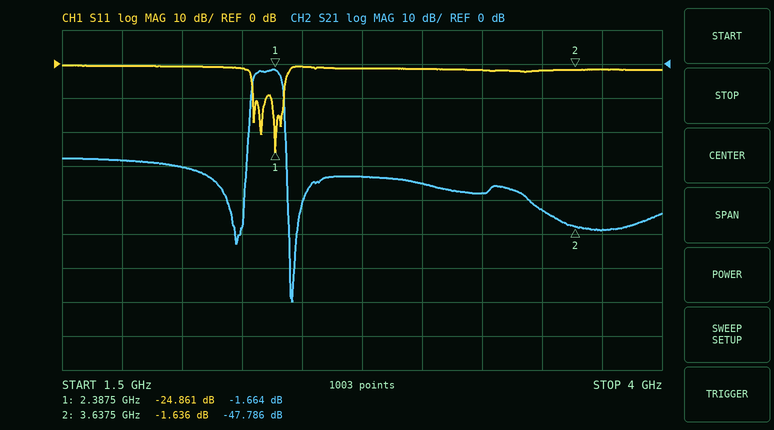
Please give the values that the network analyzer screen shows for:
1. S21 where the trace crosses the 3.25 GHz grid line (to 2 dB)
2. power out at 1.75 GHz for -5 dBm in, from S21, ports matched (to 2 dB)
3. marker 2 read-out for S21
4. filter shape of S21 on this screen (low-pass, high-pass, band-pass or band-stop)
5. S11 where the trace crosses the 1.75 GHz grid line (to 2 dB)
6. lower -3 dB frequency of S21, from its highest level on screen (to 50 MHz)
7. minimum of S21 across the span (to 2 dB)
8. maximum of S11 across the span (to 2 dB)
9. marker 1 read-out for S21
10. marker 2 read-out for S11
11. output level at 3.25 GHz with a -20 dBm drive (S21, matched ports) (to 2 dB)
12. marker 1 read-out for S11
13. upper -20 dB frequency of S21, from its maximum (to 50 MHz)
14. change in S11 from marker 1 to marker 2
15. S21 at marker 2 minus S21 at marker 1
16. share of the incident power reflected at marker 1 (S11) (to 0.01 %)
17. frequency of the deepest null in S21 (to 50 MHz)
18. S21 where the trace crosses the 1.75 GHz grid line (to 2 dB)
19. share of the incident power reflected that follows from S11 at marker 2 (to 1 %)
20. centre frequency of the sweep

-38 dB
-34 dBm
-47.786 dB
band-pass
0 dB
2.30 GHz
-70 dB
0 dB
-1.664 dB
-1.636 dB
-58 dBm
-24.861 dB
2.45 GHz
23.225 dB
-46.122 dB
0.33 %
2.45 GHz
-28 dB
69 %
2.75 GHz
